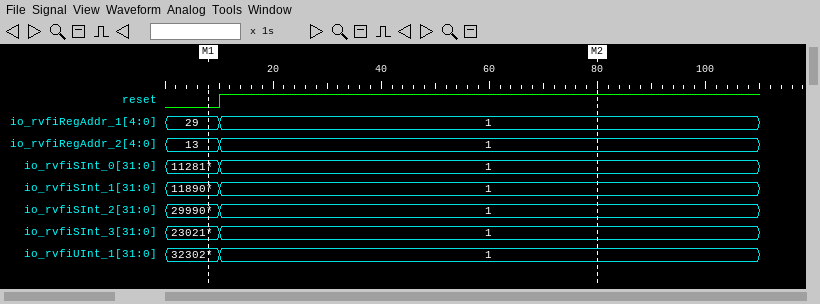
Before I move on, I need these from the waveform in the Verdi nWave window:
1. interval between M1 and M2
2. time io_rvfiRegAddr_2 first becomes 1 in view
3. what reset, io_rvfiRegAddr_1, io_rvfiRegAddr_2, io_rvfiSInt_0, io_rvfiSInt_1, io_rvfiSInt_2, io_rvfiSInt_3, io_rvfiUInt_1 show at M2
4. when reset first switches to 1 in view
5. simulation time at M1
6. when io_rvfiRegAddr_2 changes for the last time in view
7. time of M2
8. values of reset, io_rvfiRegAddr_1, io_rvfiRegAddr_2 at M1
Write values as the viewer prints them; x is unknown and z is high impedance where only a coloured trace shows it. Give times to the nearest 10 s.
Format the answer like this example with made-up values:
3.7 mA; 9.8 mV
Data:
70 s; 10 s; reset=1, io_rvfiRegAddr_1=1, io_rvfiRegAddr_2=1, io_rvfiSInt_0=1, io_rvfiSInt_1=1, io_rvfiSInt_2=1, io_rvfiSInt_3=1, io_rvfiUInt_1=1; 10 s; 10 s; 10 s; 80 s; reset=0, io_rvfiRegAddr_1=29, io_rvfiRegAddr_2=13
